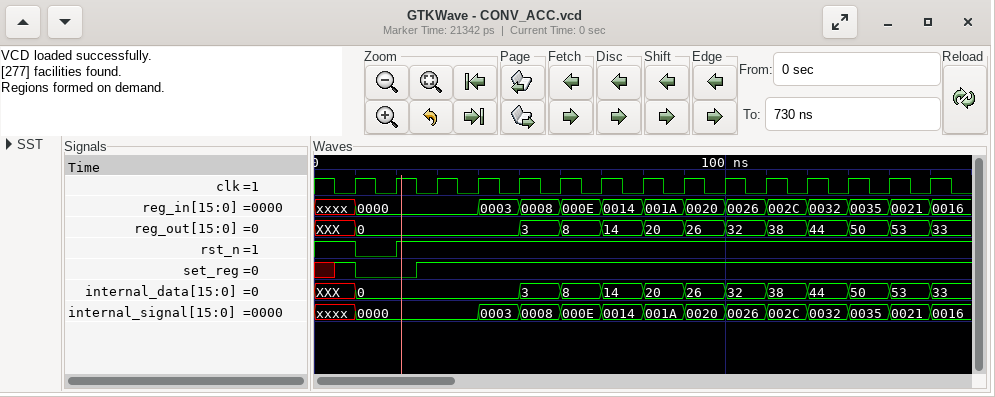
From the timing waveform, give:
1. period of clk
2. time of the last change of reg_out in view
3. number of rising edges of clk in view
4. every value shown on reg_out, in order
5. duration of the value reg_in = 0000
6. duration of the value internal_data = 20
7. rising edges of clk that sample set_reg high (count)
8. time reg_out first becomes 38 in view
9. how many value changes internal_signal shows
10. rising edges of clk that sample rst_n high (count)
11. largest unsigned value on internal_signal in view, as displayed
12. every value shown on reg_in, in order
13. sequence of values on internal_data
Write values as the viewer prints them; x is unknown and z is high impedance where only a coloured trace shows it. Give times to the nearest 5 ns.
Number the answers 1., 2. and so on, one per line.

1. 10 ns
2. 150 ns
3. 15
4. XXX, 0, 3, 8, 14, 20, 26, 32, 38, 44, 50, 53, 33
5. 30 ns
6. 10 ns
7. 14
8. 110 ns
9. 13
10. 14
11. 0035
12. xxxx, 0000, 0003, 0008, 000E, 0014, 001A, 0020, 0026, 002C, 0032, 0035, 0021, 0016
13. XXX, 0, 3, 8, 14, 20, 26, 32, 38, 44, 50, 53, 33
